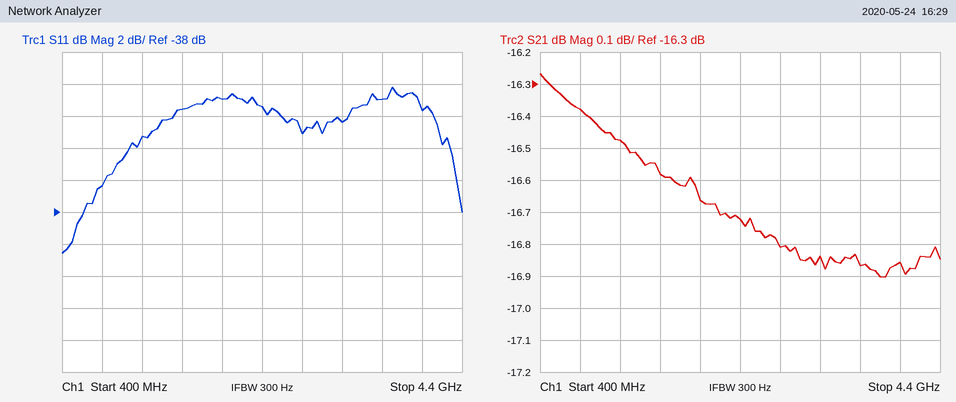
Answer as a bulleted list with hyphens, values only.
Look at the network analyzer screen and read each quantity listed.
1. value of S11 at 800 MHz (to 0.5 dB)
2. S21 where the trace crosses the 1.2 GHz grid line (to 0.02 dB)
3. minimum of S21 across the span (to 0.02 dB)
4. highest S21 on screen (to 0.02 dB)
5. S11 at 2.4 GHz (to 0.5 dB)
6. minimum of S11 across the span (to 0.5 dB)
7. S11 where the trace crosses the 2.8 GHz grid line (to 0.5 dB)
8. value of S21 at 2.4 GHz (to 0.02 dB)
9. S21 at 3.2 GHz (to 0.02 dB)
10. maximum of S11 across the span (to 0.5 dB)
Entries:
- -36.5 dB
- -16.48 dB
- -16.90 dB
- -16.26 dB
- -31.5 dB
- -40.5 dB
- -33.0 dB
- -16.72 dB
- -16.84 dB
- -30.0 dB
